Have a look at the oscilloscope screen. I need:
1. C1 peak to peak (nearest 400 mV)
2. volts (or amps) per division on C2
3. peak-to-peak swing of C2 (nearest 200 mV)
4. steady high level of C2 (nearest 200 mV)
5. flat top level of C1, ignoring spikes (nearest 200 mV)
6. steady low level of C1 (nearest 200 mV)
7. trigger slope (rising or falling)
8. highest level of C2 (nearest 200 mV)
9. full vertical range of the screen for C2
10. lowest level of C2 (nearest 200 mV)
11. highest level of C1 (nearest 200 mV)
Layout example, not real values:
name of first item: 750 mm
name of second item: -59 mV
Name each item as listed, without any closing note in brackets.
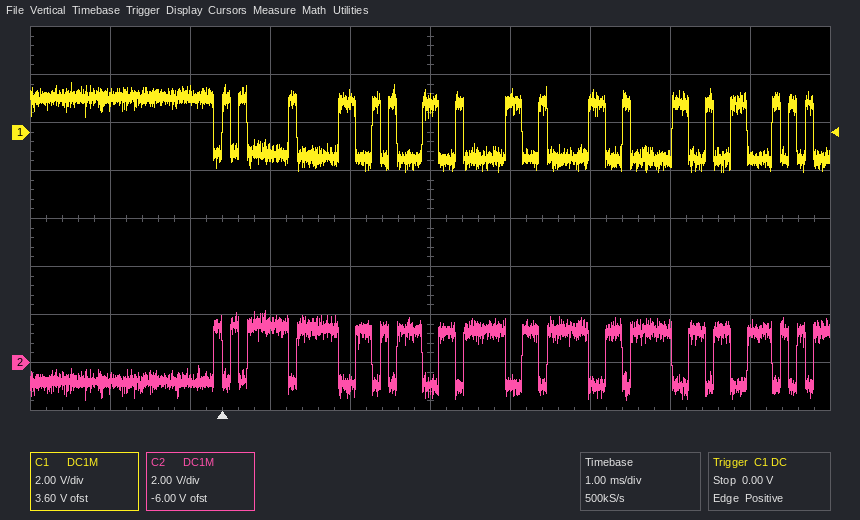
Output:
C1 peak to peak: 3.6 V
volts (or amps) per division on C2: 2 V
peak-to-peak swing of C2: 3.8 V
steady high level of C2: 1.4 V
flat top level of C1, ignoring spikes: 1.4 V
steady low level of C1: -1.0 V
trigger slope: rising
highest level of C2: 2.2 V
full vertical range of the screen for C2: 16 V
lowest level of C2: -1.6 V
highest level of C1: 2.0 V
